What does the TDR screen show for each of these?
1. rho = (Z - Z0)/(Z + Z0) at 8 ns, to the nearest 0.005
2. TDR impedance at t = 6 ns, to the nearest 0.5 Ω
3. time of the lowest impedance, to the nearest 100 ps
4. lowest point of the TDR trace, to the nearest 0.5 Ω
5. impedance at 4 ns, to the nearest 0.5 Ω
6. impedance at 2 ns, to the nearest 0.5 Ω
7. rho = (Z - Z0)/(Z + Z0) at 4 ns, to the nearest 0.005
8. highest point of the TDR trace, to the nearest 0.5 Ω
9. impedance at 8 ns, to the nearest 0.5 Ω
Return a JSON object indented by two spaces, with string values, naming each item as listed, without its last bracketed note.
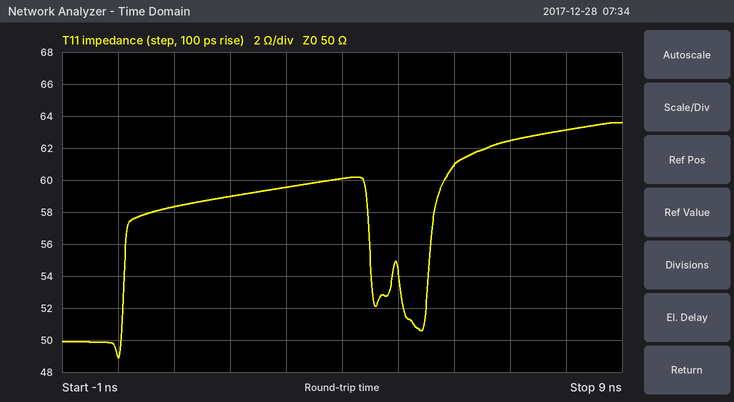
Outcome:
{
  "rho = (Z - Z0)/(Z + Z0) at 8 ns, to the nearest 0.005": "+0.115",
  "TDR impedance at t = 6 ns, to the nearest 0.5 Ω": "61.0 Ω",
  "time of the lowest impedance, to the nearest 100 ps": "0.0 ns",
  "lowest point of the TDR trace, to the nearest 0.5 Ω": "49.0 Ω",
  "impedance at 4 ns, to the nearest 0.5 Ω": "60.0 Ω",
  "impedance at 2 ns, to the nearest 0.5 Ω": "59.0 Ω",
  "rho = (Z - Z0)/(Z + Z0) at 4 ns, to the nearest 0.005": "+0.090",
  "highest point of the TDR trace, to the nearest 0.5 Ω": "63.5 Ω",
  "impedance at 8 ns, to the nearest 0.5 Ω": "63.0 Ω"
}
